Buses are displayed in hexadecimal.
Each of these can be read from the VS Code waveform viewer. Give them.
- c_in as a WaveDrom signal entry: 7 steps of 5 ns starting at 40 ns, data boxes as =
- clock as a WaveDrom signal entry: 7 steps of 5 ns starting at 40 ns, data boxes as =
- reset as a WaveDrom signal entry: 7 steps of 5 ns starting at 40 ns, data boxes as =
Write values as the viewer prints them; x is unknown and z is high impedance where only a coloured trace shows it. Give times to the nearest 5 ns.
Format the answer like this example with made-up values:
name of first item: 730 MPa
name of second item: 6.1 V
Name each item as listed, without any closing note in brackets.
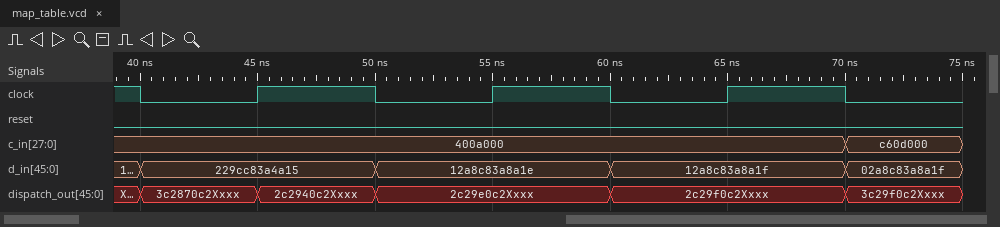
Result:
c_in as a WaveDrom signal entry: 7 steps of 5 ns starting at 40 ns, data boxes as =: {name: 'c_in', wave: '=.....=', data: '400a000 c60d000'}
clock as a WaveDrom signal entry: 7 steps of 5 ns starting at 40 ns, data boxes as =: {name: 'clock', wave: '0101010'}
reset as a WaveDrom signal entry: 7 steps of 5 ns starting at 40 ns, data boxes as =: {name: 'reset', wave: '0......'}
